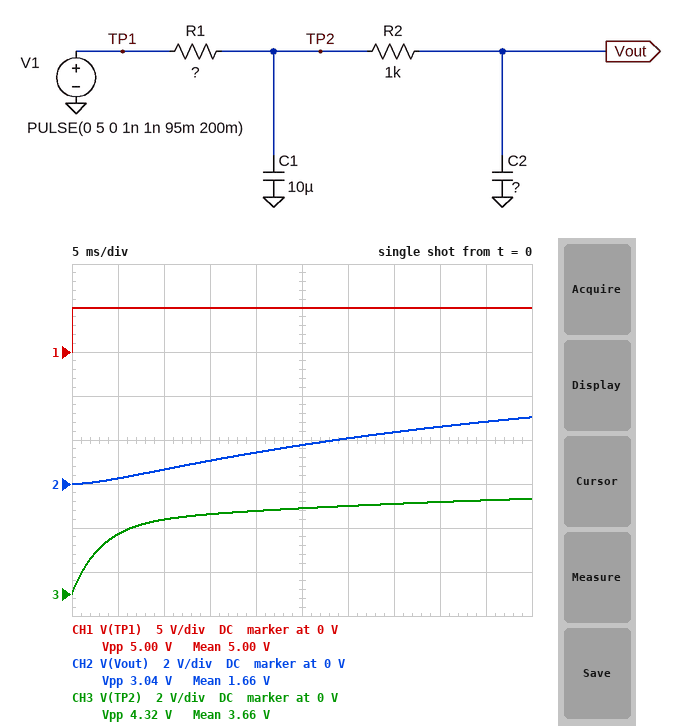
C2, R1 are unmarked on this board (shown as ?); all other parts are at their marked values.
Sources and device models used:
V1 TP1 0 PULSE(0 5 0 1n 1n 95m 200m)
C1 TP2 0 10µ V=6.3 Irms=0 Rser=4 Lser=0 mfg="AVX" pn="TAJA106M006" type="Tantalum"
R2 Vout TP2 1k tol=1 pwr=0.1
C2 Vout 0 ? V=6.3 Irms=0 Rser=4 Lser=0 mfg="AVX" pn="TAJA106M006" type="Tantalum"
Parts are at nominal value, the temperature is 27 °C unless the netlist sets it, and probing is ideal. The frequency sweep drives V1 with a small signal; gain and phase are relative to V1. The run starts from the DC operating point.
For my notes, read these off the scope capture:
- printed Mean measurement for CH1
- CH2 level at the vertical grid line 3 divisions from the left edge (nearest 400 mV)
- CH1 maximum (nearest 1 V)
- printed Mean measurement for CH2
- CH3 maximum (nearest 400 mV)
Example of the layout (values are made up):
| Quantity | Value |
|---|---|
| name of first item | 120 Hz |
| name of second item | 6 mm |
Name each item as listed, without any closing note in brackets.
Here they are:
| Quantity | Value |
|---|---|
| printed Mean measurement for CH1 | 5.00 V |
| CH2 level at the vertical grid line 3 divisions from the left edge | 1.2 V |
| CH1 maximum | 5 V |
| printed Mean measurement for CH2 | 1.66 V |
| CH3 maximum | 4.4 V |
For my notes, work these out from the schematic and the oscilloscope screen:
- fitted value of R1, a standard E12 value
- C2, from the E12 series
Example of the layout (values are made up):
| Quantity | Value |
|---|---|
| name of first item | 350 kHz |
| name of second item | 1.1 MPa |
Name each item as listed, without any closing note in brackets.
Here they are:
| Quantity | Value |
|---|---|
| fitted value of R1, a standard E12 value | 470 Ω |
| C2, from the E12 series | 33 µF |
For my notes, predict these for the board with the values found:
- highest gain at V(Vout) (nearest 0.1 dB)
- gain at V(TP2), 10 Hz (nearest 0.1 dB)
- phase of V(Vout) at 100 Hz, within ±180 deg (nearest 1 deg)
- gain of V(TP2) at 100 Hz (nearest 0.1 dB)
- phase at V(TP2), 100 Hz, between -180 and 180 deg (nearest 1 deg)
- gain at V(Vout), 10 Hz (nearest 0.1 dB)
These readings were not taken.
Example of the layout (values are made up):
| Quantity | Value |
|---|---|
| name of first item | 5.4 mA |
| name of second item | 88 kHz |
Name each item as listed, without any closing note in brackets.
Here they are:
| Quantity | Value |
|---|---|
| highest gain at V(Vout) | 0 dB |
| gain at V(TP2), 10 Hz | -3.3 dB |
| phase of V(Vout) at 100 Hz, within ±180 deg | -145 deg |
| gain of V(TP2) at 100 Hz | -10.5 dB |
| phase at V(TP2), 100 Hz, between -180 and 180 deg | -63 deg |
| gain at V(Vout), 10 Hz | -10.6 dB |
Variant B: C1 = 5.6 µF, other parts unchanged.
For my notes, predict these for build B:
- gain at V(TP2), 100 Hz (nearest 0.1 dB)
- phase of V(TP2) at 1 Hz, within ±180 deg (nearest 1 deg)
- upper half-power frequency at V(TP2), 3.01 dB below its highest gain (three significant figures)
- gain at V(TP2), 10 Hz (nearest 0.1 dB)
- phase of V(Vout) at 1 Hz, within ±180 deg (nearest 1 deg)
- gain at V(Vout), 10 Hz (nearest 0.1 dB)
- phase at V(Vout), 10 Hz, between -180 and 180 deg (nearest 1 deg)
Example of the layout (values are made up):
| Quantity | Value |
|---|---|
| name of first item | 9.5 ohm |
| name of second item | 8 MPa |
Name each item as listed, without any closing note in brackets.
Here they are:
| Quantity | Value |
|---|---|
| gain at V(TP2), 100 Hz | -7.0 dB |
| phase of V(TP2) at 1 Hz, within ±180 deg | -6 deg |
| upper half-power frequency at V(TP2), 3.01 dB below its highest gain | 9.40 Hz |
| gain at V(TP2), 10 Hz | -3.1 dB |
| phase of V(Vout) at 1 Hz, within ±180 deg | -18 deg |
| gain at V(Vout), 10 Hz | -10.3 dB |
| phase at V(Vout), 10 Hz, between -180 and 180 deg | -78 deg |
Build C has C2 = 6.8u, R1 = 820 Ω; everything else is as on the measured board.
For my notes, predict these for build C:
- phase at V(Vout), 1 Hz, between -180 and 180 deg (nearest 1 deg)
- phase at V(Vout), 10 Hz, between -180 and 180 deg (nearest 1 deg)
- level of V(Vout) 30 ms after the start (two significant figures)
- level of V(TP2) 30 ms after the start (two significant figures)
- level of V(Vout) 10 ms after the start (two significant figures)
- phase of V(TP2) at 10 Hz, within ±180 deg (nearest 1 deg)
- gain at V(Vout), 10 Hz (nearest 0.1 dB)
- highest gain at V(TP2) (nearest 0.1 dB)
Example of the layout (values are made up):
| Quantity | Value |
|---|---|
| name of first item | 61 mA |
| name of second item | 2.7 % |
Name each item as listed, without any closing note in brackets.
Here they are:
| Quantity | Value |
|---|---|
| phase at V(Vout), 1 Hz, between -180 and 180 deg | -7 deg |
| phase at V(Vout), 10 Hz, between -180 and 180 deg | -59 deg |
| level of V(Vout) 30 ms after the start | 3.9 V |
| level of V(TP2) 30 ms after the start | 4.3 V |
| level of V(Vout) 10 ms after the start | 1.6 V |
| phase of V(TP2) at 10 Hz, within ±180 deg | -36 deg |
| gain at V(Vout), 10 Hz | -3.6 dB |
| highest gain at V(TP2) | 0 dB |
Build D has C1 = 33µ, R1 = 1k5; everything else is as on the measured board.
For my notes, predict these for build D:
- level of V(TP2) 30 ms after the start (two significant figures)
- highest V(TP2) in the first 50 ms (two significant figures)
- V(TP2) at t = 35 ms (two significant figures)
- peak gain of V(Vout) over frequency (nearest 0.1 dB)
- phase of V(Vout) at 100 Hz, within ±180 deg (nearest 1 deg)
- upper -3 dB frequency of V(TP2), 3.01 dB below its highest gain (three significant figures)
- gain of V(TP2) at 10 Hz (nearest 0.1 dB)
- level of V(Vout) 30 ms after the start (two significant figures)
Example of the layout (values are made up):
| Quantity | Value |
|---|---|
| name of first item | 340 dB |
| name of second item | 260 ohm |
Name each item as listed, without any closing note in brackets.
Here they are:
| Quantity | Value |
|---|---|
| level of V(TP2) 30 ms after the start | 1.7 V |
| highest V(TP2) in the first 50 ms | 2.3 V |
| V(TP2) at t = 35 ms | 1.9 V |
| peak gain of V(Vout) over frequency | 0 dB |
| phase of V(Vout) at 100 Hz, within ±180 deg | -163 deg |
| upper -3 dB frequency of V(TP2), 3.01 dB below its highest gain | 1.44 Hz |
| gain of V(TP2) at 10 Hz | -12.7 dB |
| level of V(Vout) 30 ms after the start | 690 mV |
